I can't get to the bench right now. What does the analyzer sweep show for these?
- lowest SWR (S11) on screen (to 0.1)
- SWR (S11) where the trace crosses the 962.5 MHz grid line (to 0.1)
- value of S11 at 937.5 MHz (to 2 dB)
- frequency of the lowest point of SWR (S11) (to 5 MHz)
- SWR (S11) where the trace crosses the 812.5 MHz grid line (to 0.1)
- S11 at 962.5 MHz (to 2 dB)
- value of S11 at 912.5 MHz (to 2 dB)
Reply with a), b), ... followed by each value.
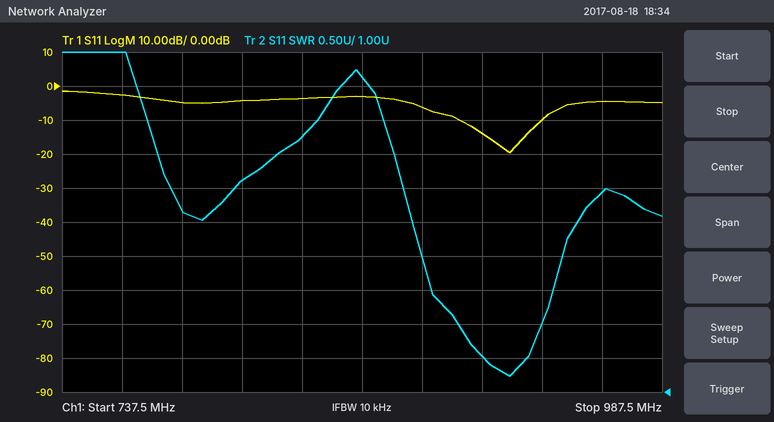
a) 1.2
b) 3.9
c) -10 dB
d) 925 MHz
e) 4.1
f) -4 dB
g) -14 dB
